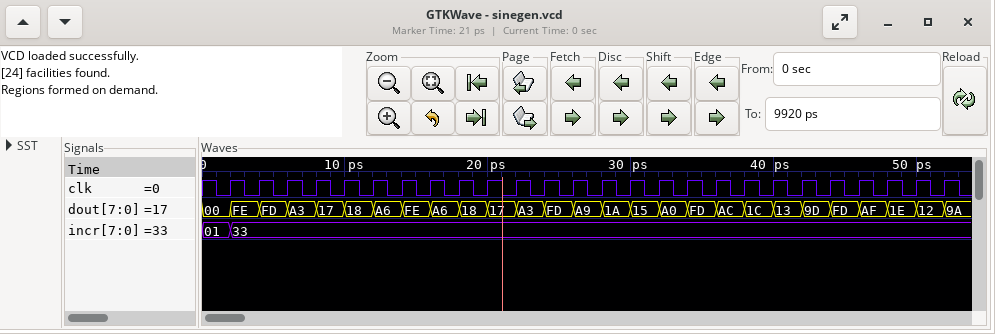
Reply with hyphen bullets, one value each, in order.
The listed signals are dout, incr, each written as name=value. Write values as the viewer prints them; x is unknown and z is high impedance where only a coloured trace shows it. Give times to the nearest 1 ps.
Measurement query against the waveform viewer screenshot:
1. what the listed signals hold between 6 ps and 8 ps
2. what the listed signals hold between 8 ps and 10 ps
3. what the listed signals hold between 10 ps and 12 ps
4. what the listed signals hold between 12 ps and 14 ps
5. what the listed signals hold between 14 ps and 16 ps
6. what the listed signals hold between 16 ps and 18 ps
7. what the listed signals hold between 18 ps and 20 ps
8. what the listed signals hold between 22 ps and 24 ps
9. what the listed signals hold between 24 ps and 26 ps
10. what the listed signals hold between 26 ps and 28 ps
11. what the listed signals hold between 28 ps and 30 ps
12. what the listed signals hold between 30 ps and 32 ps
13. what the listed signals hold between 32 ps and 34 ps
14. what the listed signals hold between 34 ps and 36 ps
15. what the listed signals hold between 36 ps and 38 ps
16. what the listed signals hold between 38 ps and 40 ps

- dout=A3, incr=33
- dout=17, incr=33
- dout=18, incr=33
- dout=A6, incr=33
- dout=FE, incr=33
- dout=A6, incr=33
- dout=18, incr=33
- dout=A3, incr=33
- dout=FD, incr=33
- dout=A9, incr=33
- dout=1A, incr=33
- dout=15, incr=33
- dout=A0, incr=33
- dout=FD, incr=33
- dout=AC, incr=33
- dout=1C, incr=33
